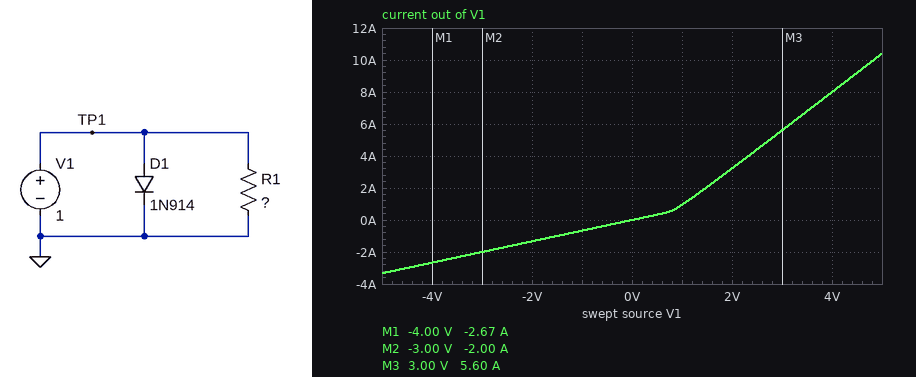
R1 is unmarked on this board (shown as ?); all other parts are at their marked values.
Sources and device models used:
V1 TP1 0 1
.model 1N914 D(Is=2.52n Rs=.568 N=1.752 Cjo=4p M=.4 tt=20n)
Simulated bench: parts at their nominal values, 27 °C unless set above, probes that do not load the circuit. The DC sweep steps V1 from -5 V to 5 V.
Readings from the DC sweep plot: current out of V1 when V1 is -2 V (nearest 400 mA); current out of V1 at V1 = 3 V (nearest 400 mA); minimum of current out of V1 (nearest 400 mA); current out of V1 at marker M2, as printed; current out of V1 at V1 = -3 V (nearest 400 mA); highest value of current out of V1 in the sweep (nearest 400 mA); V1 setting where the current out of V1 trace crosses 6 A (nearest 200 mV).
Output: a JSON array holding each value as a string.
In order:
["-1.2 A", "5.6 A", "-3.2 A", "-2.00 A", "-2.0 A", "10.4 A", "3.2 V"]
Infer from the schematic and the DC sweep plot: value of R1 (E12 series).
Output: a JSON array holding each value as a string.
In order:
["1.5 Ω"]
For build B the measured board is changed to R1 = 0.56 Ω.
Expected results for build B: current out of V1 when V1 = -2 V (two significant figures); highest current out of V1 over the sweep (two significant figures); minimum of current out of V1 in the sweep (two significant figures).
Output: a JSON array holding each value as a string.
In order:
["-3.6 A", "16 A", "-8.9 A"]
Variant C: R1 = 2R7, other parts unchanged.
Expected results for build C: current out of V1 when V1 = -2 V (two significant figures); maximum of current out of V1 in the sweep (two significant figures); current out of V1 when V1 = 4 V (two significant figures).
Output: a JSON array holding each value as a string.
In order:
["-740 mA", "8.9 A", "6.8 A"]
